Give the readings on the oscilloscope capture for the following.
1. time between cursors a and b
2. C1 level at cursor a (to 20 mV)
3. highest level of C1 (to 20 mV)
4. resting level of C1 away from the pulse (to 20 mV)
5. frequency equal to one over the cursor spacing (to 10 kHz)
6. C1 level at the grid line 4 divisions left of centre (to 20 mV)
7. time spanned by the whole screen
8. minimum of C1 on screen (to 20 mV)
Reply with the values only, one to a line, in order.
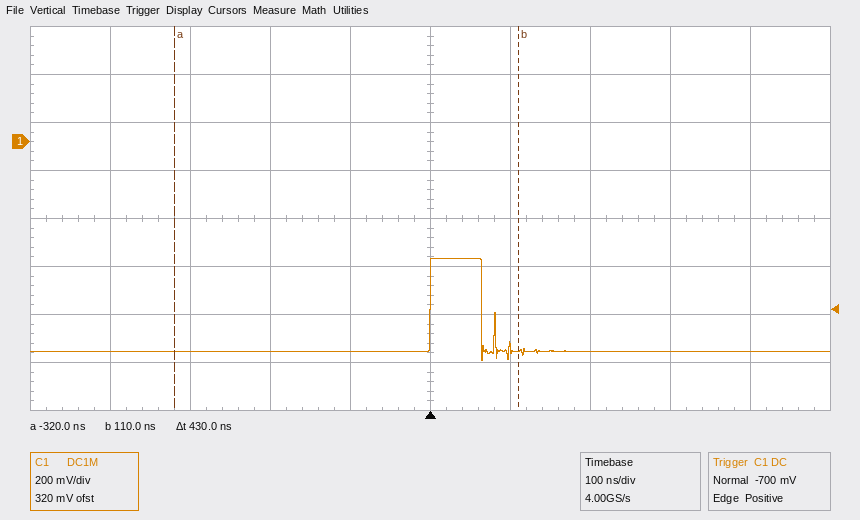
430 ns
-880 mV
-480 mV
-880 mV
2.33 MHz
-880 mV
1 µs
-920 mV
